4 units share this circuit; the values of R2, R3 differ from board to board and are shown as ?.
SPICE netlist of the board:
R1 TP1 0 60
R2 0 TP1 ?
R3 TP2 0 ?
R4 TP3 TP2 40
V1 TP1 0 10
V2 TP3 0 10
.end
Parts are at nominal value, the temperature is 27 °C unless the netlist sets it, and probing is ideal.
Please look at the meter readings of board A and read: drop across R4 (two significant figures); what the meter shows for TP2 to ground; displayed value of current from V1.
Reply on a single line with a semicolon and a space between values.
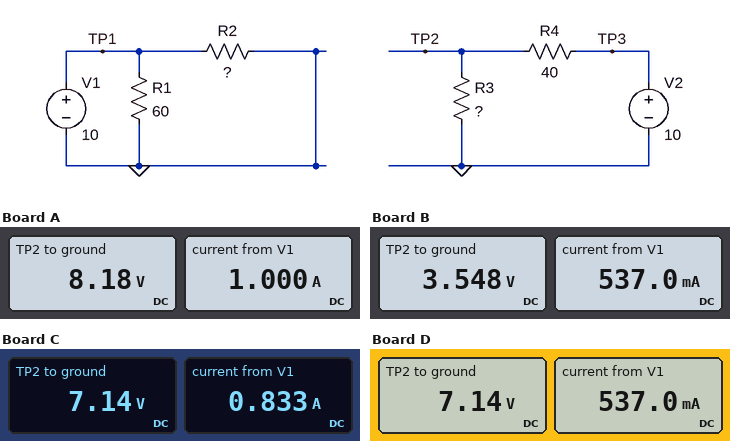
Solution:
1.8 V; 8.18 V; 1.000 A
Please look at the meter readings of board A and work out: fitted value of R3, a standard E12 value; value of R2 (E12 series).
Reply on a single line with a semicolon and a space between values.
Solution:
180 Ω; 12 Ω
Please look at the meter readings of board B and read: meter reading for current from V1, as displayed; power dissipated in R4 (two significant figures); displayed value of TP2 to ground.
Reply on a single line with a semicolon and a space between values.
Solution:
537.0 mA; 1.0 W; 3.548 V
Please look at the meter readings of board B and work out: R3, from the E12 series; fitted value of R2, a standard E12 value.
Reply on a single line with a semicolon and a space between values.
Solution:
22 Ω; 27 Ω
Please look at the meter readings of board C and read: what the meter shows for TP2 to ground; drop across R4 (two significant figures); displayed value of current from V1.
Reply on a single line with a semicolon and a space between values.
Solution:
7.14 V; 2.9 V; 0.833 A
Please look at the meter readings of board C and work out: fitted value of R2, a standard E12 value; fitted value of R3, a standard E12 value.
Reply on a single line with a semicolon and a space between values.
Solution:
15 Ω; 100 Ω
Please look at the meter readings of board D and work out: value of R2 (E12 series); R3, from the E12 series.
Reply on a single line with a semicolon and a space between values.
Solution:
27 Ω; 100 Ω
